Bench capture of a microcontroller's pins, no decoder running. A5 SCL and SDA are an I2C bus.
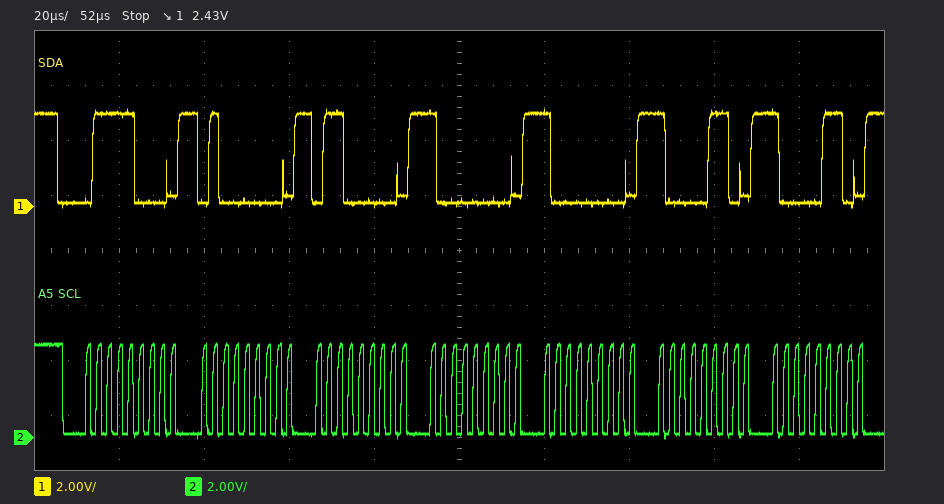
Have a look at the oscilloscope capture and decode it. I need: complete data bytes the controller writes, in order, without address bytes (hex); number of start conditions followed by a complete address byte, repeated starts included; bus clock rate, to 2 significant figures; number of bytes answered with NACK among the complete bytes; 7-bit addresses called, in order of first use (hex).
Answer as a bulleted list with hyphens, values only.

- 40 60 80 80 86 86
- 1
- 400 kHz
- 0
- 0x3C
